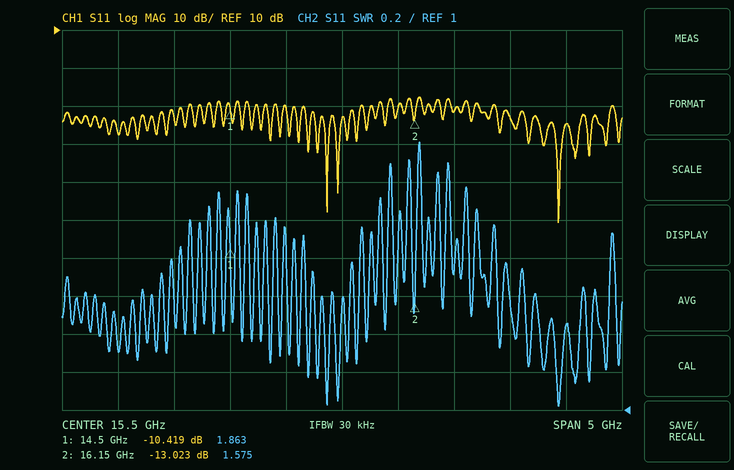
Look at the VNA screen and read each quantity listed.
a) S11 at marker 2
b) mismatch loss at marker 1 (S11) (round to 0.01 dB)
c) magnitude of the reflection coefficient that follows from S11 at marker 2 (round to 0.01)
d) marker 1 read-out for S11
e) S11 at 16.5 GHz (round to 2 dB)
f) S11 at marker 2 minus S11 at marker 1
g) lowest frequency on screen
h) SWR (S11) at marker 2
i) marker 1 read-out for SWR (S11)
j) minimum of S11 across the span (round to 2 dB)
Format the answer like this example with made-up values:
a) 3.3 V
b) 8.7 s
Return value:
a) -13.023 dB
b) 0.41 dB
c) 0.22
d) -10.419 dB
e) -12 dB
f) -2.604 dB
g) 13 GHz
h) 1.575
i) 1.863
j) -40 dB
